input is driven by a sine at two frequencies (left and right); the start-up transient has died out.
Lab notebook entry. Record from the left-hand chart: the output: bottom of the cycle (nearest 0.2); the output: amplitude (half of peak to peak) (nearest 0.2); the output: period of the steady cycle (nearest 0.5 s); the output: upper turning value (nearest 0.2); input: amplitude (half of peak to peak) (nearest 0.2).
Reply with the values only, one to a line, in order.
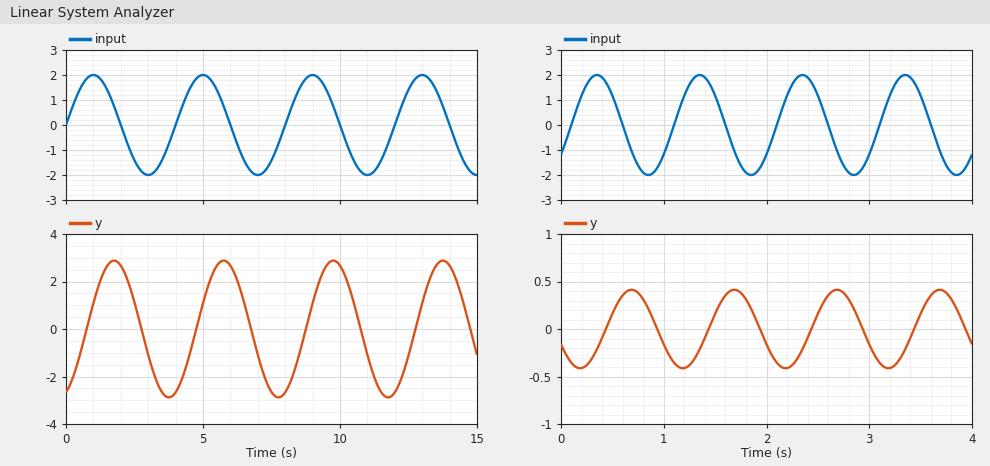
-2.8
2.8
4.0 s
2.8
2.0
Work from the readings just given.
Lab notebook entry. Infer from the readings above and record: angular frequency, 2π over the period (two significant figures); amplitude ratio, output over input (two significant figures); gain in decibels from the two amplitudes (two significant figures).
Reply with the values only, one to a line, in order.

1.6 rad/s
1.4
2.9 dB
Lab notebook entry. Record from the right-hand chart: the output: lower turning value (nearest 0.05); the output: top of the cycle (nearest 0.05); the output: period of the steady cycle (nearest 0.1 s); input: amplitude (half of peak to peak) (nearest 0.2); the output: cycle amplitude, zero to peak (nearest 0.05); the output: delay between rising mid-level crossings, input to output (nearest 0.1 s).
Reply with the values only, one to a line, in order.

-0.40
0.40
1.0 s
2.0
0.40
0.3 s
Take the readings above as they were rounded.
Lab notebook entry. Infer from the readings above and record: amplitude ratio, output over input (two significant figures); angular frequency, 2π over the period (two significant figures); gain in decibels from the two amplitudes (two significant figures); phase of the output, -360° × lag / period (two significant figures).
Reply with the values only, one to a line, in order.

0.20
6.3 rad/s
-14 dB
-110°
